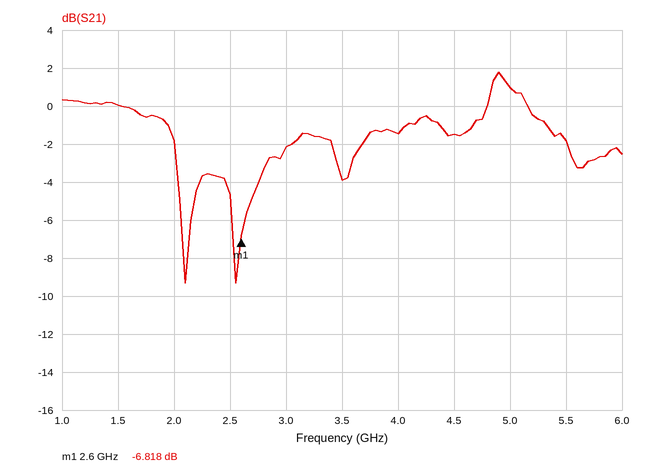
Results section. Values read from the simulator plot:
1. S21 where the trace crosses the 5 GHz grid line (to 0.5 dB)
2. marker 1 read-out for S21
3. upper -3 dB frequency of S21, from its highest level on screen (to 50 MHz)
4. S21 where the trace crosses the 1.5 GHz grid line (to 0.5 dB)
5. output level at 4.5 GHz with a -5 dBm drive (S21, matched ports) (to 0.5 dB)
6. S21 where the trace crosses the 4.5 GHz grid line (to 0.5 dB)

1.0 dB
-6.818 dB
5.35 GHz
0.0 dB
-6.5 dBm
-1.5 dB
